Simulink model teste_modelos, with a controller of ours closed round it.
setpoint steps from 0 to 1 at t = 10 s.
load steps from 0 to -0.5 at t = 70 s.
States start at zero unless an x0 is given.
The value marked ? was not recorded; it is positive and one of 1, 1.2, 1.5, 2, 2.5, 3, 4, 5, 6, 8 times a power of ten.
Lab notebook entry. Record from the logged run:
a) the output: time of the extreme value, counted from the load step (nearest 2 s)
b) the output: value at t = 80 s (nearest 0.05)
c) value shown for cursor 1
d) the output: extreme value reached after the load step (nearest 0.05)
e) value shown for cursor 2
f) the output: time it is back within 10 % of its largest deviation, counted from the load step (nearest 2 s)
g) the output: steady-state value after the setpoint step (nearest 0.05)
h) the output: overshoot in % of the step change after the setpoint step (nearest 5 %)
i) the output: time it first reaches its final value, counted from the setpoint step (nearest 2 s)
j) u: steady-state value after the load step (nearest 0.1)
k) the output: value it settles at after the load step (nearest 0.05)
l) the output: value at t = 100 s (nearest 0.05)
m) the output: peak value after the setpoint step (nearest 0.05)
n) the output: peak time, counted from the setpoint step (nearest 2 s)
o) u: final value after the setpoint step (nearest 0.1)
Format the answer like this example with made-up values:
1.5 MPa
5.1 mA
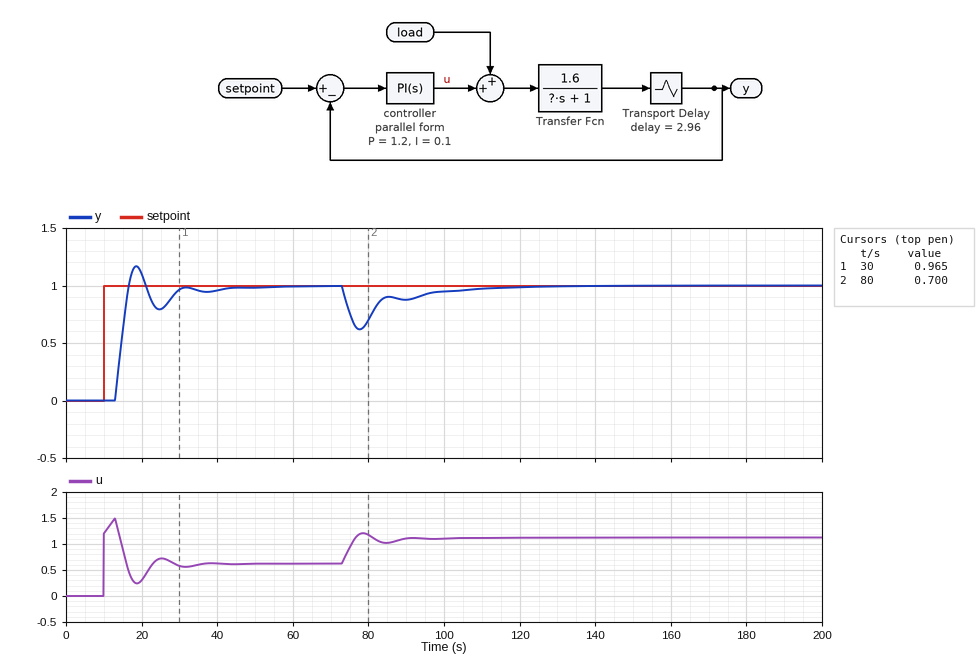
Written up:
8 s
0.70
0.965
0.60
0.700
36 s
1.00
15 %
6 s
1.1
1.00
0.95
1.15
8 s
0.6
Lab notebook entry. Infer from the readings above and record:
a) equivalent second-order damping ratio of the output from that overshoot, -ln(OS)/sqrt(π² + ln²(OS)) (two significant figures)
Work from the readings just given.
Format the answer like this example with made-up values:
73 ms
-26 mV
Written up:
0.52
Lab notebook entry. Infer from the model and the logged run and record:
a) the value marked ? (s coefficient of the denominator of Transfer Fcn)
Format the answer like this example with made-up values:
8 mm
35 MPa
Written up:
6
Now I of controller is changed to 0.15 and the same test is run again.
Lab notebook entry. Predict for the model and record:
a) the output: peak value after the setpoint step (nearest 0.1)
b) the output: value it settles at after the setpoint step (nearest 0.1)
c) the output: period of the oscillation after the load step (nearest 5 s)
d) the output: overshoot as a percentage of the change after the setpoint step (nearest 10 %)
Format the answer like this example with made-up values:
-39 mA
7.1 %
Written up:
1.3
1.0
15 s
30 %
